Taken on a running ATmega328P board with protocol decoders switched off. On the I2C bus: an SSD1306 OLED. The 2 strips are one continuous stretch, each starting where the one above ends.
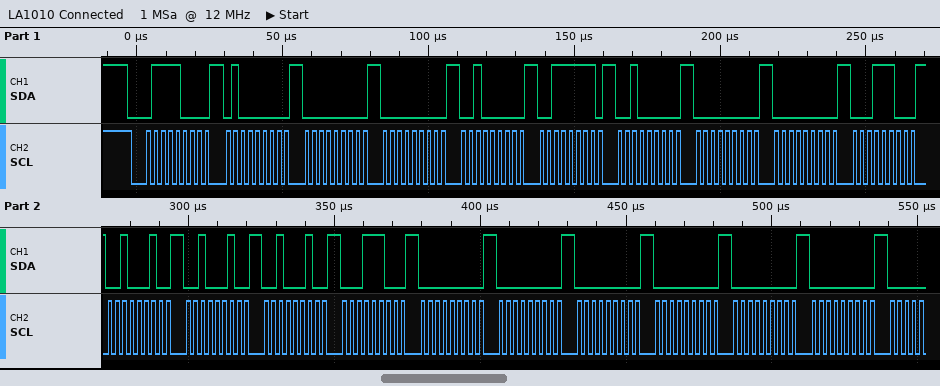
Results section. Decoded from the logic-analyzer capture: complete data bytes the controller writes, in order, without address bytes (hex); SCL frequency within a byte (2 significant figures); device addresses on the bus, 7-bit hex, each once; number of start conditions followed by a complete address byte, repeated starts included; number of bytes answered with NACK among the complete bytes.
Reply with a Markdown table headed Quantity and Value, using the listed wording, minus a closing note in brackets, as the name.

| Quantity | Value |
|---|---|
| complete data bytes the controller writes, in order, without address bytes | 40 00 00 20 3F 20 00 00 1C 22 22 22 1C 00 00 00 00 00 00 |
| SCL frequency within a byte | 400 kHz |
| device addresses on the bus, 7-bit hex, each once | 0x3C |
| number of start conditions followed by a complete address byte, repeated starts included | 1 |
| number of bytes answered with NACK among the complete bytes | 0 |
